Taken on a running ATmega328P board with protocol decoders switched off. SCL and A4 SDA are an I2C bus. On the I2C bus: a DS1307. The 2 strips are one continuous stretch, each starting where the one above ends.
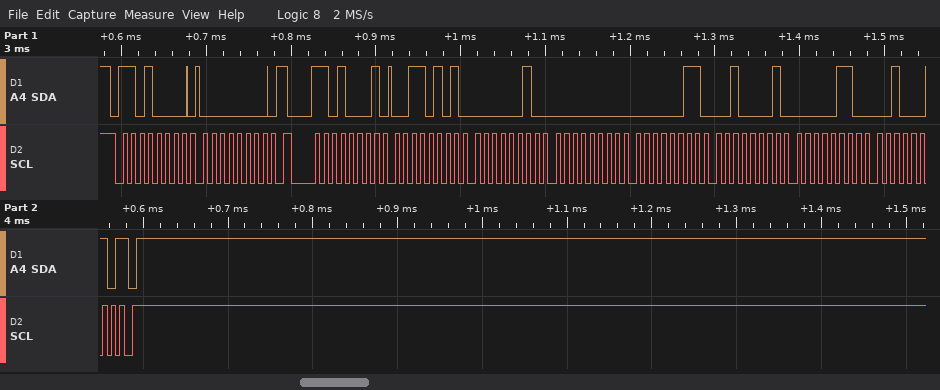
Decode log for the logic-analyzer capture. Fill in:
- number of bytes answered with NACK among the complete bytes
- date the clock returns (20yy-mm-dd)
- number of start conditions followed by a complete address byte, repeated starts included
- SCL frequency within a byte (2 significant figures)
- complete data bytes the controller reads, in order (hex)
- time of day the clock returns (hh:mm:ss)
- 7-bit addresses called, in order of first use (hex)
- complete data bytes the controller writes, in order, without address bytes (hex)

1
2022-06-21
2
100 kHz
35 02 00 03 21 06 22
00:02:35
0x68
00
